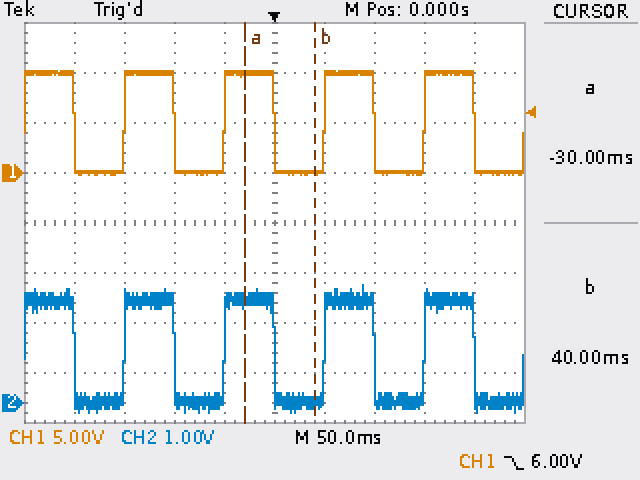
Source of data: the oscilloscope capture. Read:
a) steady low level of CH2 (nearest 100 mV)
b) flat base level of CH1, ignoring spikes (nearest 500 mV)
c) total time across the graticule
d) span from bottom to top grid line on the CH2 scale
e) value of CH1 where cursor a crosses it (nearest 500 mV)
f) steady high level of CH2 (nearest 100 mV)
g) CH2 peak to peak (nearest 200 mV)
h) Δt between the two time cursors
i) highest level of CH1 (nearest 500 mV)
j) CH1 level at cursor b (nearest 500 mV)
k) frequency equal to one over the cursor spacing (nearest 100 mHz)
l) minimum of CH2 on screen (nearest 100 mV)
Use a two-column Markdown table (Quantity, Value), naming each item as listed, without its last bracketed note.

| Quantity | Value |
|---|---|
| steady low level of CH2 | 0.0 V |
| flat base level of CH1, ignoring spikes | 0.0 V |
| total time across the graticule | 500 ms |
| span from bottom to top grid line on the CH2 scale | 8 V |
| value of CH1 where cursor a crosses it | 10.0 V |
| steady high level of CH2 | 2.0 V |
| CH2 peak to peak | 2.6 V |
| Δt between the two time cursors | 70 ms |
| highest level of CH1 | 10.0 V |
| CH1 level at cursor b | 0.0 V |
| frequency equal to one over the cursor spacing | 14.3 Hz |
| minimum of CH2 on screen | -200 mV |
